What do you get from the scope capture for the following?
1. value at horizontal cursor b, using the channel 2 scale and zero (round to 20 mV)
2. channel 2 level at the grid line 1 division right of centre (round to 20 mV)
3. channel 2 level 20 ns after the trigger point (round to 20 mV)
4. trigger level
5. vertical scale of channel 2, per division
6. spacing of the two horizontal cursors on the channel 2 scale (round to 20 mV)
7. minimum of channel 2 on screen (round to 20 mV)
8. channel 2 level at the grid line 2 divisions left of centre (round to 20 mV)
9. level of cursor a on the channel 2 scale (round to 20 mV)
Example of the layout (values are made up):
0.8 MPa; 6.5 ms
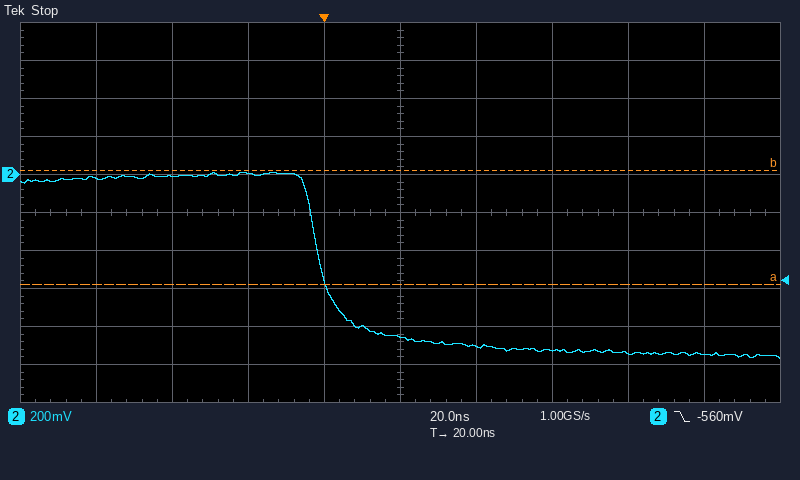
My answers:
20 mV; -900 mV; -860 mV; -560 mV; 200 mV; 600 mV; -960 mV; 0 mV; -580 mV
